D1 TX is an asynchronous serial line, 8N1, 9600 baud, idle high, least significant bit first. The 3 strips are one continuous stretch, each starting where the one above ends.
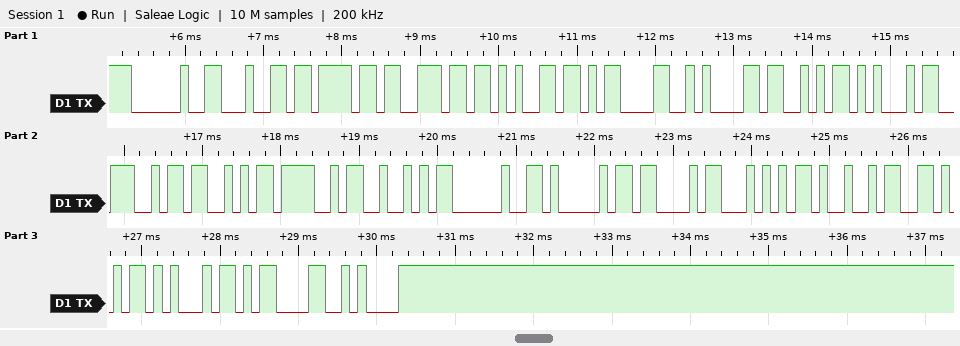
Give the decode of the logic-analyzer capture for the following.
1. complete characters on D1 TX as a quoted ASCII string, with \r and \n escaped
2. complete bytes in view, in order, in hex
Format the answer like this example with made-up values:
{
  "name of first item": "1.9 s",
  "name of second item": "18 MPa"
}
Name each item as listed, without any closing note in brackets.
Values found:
{
  "complete characters on D1 TX as a quoted ASCII string, with \\r and \\n escaped": "\" done\\r\\nSENSOR ACTIVE\\r\\n\"",
  "complete bytes in view, in order, in hex": "20 64 6F 6E 65 0D 0A 53 45 4E 53 4F 52 20 41 43 54 49 56 45 0D 0A"
}
